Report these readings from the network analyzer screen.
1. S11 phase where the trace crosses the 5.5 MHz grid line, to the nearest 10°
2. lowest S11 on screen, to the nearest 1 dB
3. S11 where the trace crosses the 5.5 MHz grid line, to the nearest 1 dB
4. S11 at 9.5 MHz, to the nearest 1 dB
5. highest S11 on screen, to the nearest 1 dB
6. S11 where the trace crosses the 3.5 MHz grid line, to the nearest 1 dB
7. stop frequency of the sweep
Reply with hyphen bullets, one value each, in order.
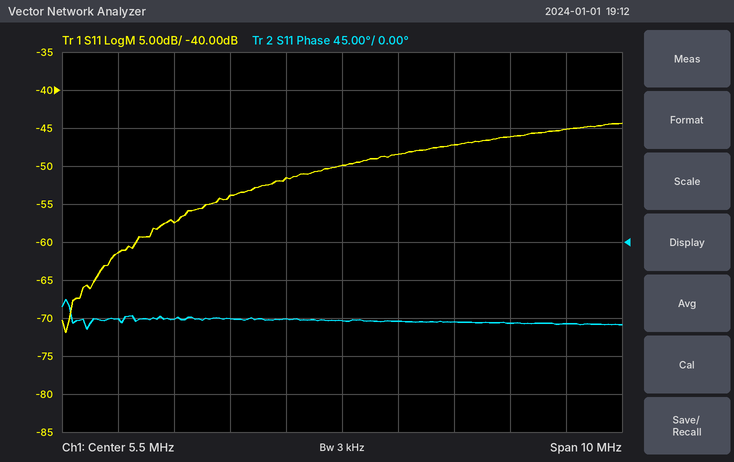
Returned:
- -90°
- -72 dB
- -50 dB
- -45 dB
- -44 dB
- -54 dB
- 10.5 MHz
